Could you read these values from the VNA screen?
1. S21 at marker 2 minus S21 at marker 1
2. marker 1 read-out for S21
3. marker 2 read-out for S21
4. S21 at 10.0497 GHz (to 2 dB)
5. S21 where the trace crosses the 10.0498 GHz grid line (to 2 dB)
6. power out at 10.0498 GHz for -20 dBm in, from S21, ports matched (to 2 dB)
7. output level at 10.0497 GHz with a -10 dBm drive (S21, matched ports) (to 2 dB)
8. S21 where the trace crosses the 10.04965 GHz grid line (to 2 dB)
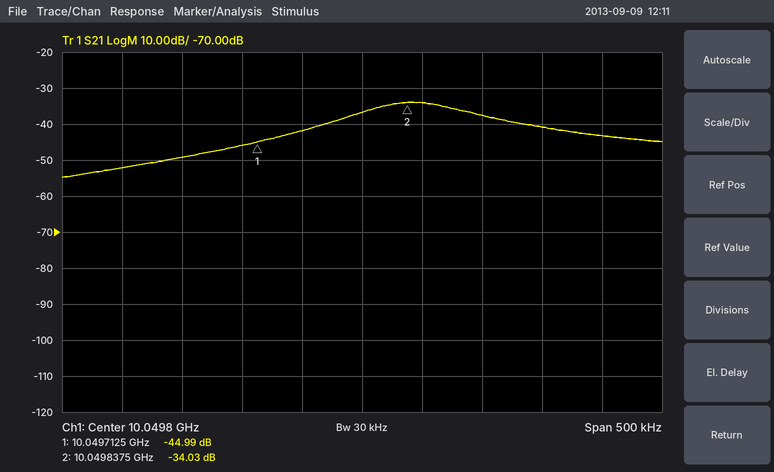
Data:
10.96 dB
-44.99 dB
-34.03 dB
-46 dB
-36 dB
-56 dBm
-56 dBm
-50 dB
